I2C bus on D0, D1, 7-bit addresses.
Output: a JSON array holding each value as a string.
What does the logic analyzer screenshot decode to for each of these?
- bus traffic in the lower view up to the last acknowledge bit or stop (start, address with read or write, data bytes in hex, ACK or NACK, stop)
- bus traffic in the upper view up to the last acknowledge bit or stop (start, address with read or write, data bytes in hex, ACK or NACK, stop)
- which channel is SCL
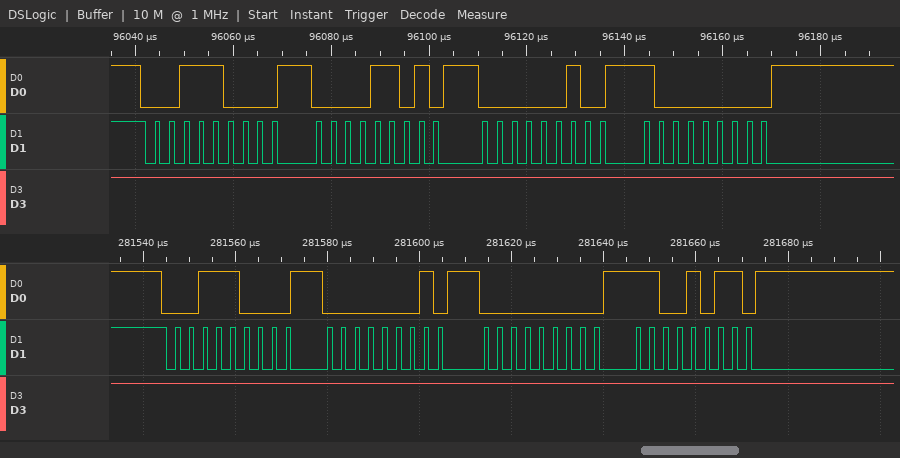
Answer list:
["start, address 1C write ACK, 01 ACK, 00 ACK, CB ACK", "start, address 1C write ACK, 0D ACK, 02 ACK, 80 ACK", "D1"]
